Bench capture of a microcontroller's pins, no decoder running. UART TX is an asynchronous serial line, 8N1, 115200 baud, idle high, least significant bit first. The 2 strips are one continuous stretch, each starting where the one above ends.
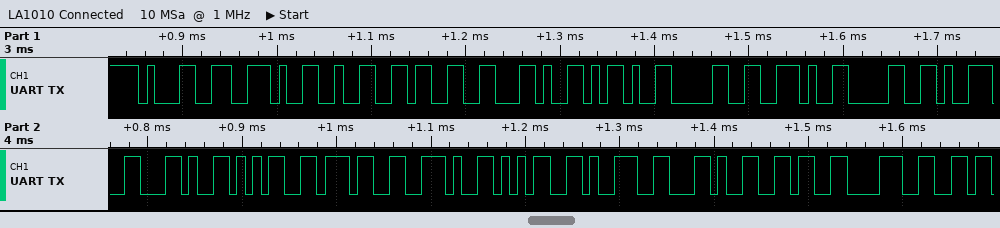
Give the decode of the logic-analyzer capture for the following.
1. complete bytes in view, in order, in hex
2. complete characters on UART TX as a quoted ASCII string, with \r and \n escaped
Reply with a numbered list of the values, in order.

1. 0x31 0x2E 0x32 0x33 0x2C 0x2D 0x30 0x2E 0x30 0x39 0x2C 0x35 0x37 0x2E 0x35 0x39 0x2C 0x36 0x38
2. "1.23,-0.09,57.59,68"
